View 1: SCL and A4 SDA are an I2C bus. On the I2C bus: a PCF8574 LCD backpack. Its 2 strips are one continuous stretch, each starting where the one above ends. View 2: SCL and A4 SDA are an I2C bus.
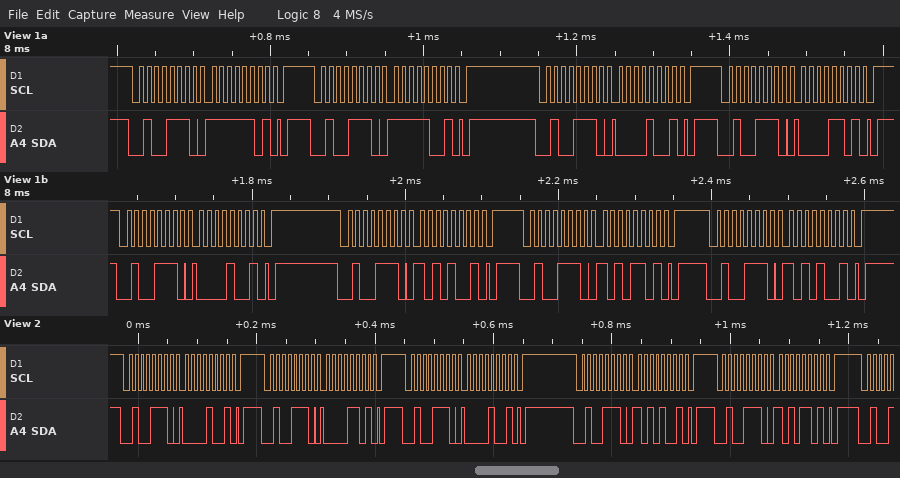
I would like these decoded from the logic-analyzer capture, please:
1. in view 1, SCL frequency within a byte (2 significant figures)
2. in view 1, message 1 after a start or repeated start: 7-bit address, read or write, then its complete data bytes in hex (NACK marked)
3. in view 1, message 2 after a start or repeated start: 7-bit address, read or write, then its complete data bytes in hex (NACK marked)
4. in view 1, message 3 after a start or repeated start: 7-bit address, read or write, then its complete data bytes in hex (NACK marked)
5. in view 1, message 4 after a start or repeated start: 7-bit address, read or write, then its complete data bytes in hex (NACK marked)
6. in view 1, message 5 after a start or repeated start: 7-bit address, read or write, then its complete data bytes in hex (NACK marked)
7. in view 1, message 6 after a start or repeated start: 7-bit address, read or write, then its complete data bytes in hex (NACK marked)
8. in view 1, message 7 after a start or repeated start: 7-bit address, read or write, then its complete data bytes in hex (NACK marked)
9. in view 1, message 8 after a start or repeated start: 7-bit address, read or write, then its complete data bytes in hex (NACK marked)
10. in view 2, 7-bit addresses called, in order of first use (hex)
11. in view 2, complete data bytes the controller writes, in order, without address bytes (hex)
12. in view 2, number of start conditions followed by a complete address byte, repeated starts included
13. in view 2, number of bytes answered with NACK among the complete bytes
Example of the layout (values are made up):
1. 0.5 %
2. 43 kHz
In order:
1. 100 kHz
2. 0x27 write: FD
3. 0x27 write: F9
4. 0x27 write: 09
5. 0x27 write: 0D
6. 0x27 write: 09
7. 0x27 write: A9
8. 0x27 write: AD
9. 0x27 write: A9
10. 0x27
11. 09 0D 09 A9 AD
12. 5
13. 0
